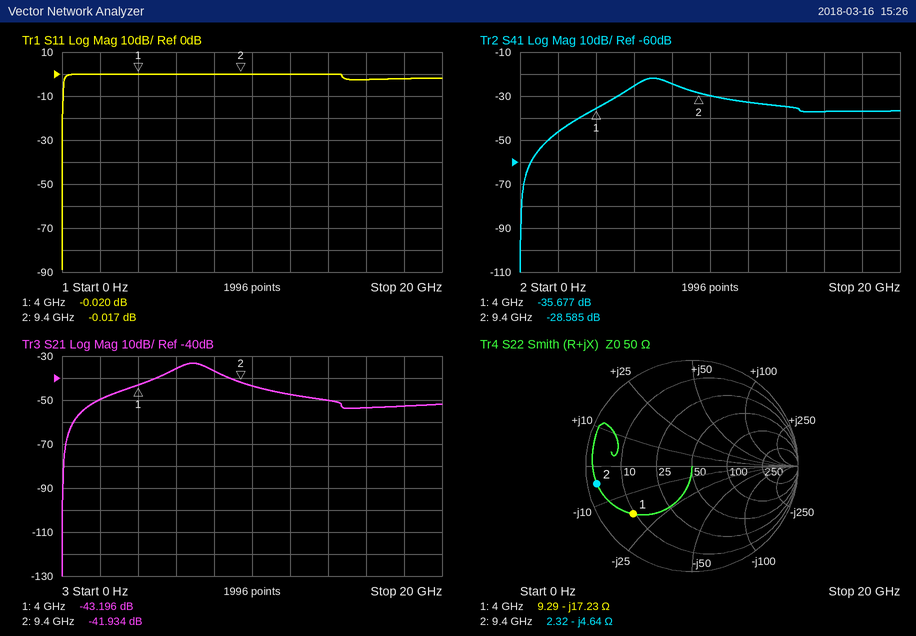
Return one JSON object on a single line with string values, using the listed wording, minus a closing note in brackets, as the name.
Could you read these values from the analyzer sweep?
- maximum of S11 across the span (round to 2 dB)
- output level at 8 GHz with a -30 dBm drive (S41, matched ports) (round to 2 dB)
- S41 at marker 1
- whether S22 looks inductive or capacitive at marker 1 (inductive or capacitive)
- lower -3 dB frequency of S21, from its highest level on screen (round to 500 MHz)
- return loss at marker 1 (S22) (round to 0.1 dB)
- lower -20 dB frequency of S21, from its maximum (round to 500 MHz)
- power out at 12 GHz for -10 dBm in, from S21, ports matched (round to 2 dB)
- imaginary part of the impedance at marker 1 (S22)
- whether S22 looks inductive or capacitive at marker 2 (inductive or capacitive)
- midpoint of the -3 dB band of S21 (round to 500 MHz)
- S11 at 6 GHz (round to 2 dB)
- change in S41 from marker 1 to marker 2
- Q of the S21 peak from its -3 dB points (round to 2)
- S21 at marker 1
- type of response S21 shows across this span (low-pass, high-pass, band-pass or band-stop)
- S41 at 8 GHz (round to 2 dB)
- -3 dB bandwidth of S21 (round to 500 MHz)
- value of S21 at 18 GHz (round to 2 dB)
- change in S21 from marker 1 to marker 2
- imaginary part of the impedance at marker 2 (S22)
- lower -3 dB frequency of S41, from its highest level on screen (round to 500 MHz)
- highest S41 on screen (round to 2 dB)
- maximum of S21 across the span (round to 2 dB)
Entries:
{"maximum of S11 across the span": "0 dB", "output level at 8 GHz with a -30 dBm drive (S41, matched ports)": "-54 dBm", "S41 at marker 1": "-35.677 dB", "whether S22 looks inductive or capacitive at marker 1": "capacitive", "lower -3 dB frequency of S21, from its highest level on screen": "6.0 GHz", "return loss at marker 1 (S22)": "2.9 dB", "lower -20 dB frequency of S21, from its maximum": "1.5 GHz", "power out at 12 GHz for -10 dBm in, from S21, ports matched": "-58 dBm", "imaginary part of the impedance at marker 1": "-17.23 Ω", "whether S22 looks inductive or capacitive at marker 2": "capacitive", "midpoint of the -3 dB band of S21": "7.0 GHz", "S11 at 6 GHz": "0 dB", "change in S41 from marker 1 to marker 2": "7.092 dB", "Q of the S21 peak from its -3 dB points": "4", "S21 at marker 1": "-43.196 dB", "type of response S21 shows across this span": "band-pass", "S41 at 8 GHz": "-24 dB", "-3 dB bandwidth of S21": "2.0 GHz", "value of S21 at 18 GHz": "-52 dB", "change in S21 from marker 1 to marker 2": "1.262 dB", "imaginary part of the impedance at marker 2": "-4.64 Ω", "lower -3 dB frequency of S41, from its highest level on screen": "6.0 GHz", "highest S41 on screen": "-22 dB", "maximum of S21 across the span": "-34 dB"}
